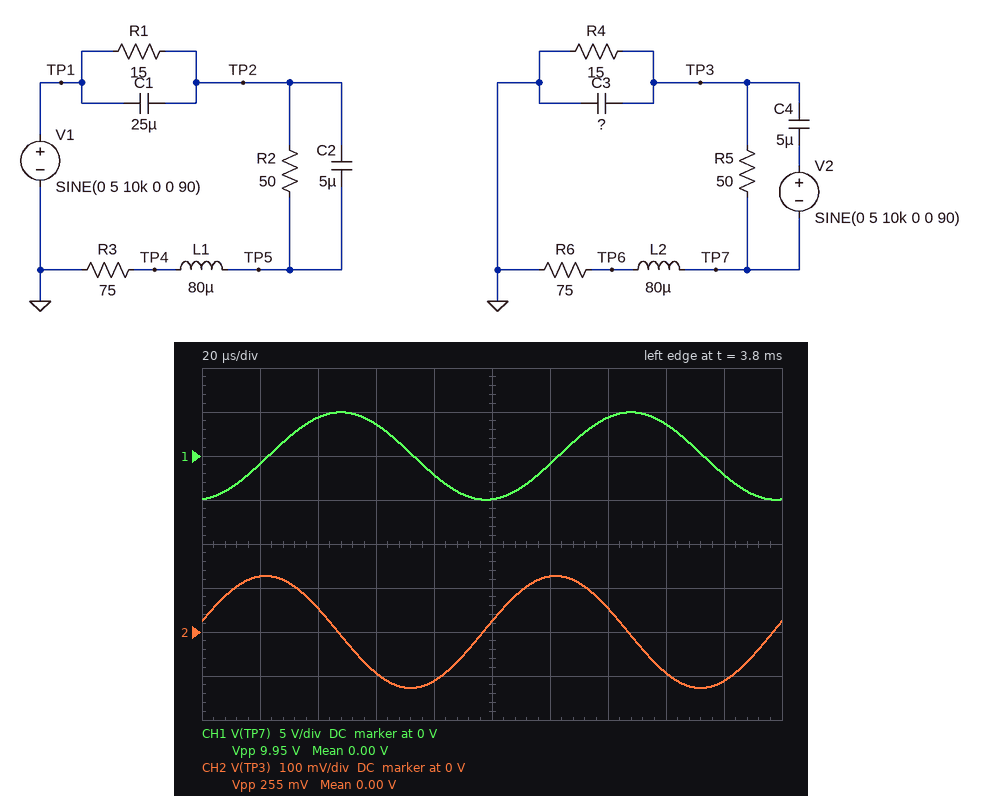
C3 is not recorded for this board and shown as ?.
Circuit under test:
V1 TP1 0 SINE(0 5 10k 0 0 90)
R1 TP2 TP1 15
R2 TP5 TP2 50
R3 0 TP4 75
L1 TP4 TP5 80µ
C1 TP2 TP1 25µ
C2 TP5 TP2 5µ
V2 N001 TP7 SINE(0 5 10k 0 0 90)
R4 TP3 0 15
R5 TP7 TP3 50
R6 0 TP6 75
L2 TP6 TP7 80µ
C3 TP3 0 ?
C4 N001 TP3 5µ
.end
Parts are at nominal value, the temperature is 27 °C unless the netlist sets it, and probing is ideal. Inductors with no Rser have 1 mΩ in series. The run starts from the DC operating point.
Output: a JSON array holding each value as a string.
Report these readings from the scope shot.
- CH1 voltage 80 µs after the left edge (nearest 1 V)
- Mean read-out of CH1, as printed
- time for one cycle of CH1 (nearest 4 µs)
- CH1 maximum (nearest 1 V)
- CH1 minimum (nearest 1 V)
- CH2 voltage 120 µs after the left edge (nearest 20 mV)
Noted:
["-2 V", "0.00 V", "100 µs", "5 V", "-5 V", "120 mV"]
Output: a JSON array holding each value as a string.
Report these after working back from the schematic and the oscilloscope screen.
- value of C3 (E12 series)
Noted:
["8.2 µF"]
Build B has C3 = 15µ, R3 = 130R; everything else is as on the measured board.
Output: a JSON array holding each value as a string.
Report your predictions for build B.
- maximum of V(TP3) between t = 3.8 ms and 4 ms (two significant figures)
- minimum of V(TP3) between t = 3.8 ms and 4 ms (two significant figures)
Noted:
["70 mV", "-70 mV"]
